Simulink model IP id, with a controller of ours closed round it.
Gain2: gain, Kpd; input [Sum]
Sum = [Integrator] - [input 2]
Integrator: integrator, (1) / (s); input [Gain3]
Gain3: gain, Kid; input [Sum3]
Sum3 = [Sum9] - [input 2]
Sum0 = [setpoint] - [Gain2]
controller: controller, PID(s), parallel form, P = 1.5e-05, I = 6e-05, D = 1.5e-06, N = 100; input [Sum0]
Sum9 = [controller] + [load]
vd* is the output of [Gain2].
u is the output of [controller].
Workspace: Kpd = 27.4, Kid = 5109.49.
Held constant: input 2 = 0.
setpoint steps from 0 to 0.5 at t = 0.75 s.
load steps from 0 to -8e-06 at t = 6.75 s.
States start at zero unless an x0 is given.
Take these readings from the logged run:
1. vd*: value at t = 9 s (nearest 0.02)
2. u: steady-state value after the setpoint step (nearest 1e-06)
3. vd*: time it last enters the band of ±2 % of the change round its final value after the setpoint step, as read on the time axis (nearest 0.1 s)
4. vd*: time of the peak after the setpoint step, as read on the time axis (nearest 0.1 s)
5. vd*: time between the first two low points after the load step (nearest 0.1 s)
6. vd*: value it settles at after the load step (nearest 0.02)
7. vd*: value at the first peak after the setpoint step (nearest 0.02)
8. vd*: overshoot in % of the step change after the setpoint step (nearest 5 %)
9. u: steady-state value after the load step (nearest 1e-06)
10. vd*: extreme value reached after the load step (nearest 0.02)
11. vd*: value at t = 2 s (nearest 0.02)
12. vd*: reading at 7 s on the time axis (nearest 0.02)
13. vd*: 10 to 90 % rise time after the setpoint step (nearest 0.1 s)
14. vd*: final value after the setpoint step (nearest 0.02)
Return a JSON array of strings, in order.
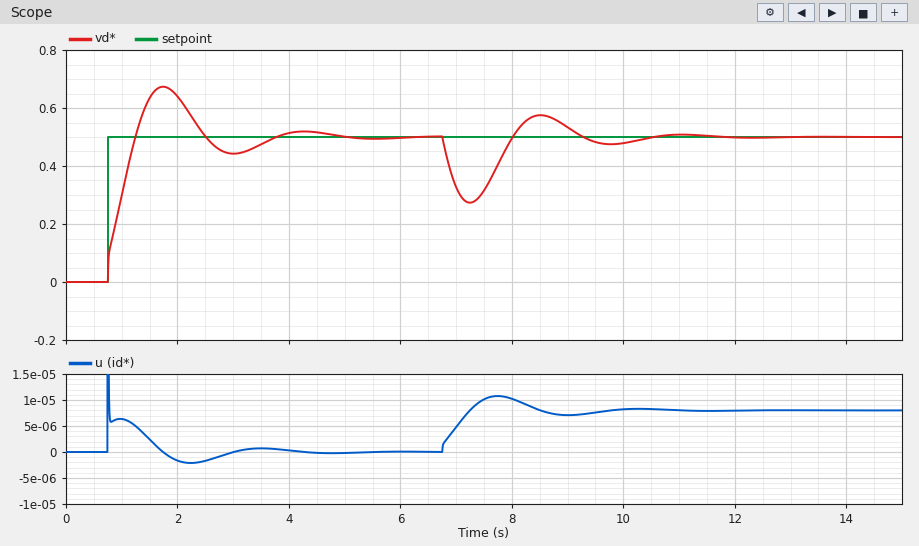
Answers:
["0.54", "0.000000", "4.7 s", "1.7 s", "2.5 s", "0.50", "0.68", "35 %", "0.000008", "0.28", "0.64", "0.32", "0.4 s", "0.50"]
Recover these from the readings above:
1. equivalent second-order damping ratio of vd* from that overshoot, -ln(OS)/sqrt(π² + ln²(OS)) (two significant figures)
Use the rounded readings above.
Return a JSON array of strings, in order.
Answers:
["0.32"]
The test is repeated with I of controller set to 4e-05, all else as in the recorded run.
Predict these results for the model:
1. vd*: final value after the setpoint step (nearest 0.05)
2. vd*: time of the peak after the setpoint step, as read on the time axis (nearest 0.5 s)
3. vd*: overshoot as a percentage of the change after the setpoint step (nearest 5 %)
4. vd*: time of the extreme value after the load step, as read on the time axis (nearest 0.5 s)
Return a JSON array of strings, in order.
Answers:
["0.50", "2.0 s", "30 %", "7.5 s"]
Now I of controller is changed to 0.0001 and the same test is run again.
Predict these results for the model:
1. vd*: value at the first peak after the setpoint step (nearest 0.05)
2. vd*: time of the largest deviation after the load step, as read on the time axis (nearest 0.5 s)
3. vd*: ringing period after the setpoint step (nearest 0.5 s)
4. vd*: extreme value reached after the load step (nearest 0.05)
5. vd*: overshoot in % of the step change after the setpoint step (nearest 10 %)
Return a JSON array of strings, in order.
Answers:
["0.70", "7.0 s", "2.0 s", "0.30", "40 %"]
